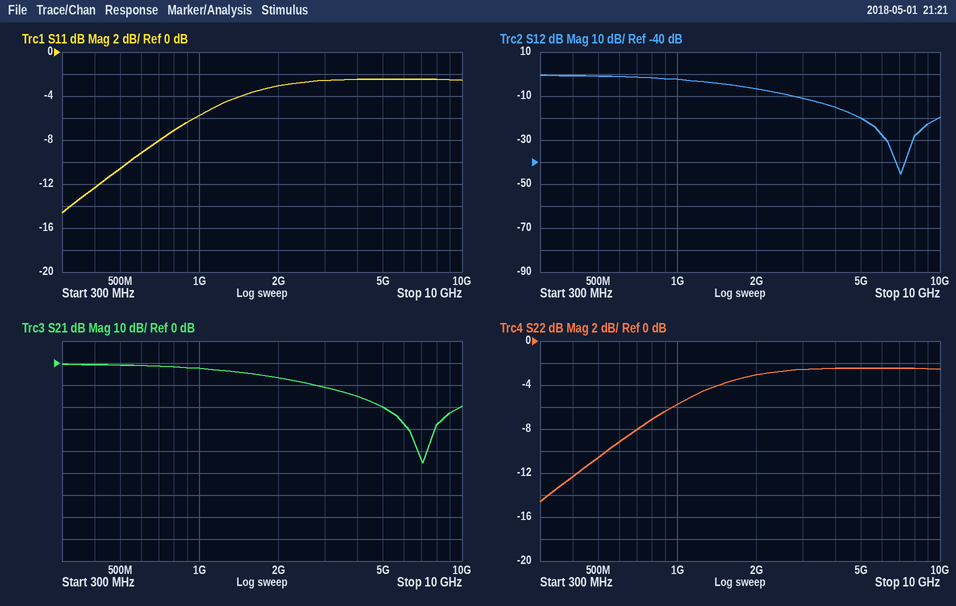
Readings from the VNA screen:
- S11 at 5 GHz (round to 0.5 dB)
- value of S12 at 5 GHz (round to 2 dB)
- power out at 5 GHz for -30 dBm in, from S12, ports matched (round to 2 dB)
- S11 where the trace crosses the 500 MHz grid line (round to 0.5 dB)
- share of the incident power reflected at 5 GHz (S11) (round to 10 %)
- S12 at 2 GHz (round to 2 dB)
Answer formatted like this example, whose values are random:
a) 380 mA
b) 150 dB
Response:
a) -2.5 dB
b) -20 dB
c) -50 dBm
d) -10.5 dB
e) 60 %
f) -6 dB
